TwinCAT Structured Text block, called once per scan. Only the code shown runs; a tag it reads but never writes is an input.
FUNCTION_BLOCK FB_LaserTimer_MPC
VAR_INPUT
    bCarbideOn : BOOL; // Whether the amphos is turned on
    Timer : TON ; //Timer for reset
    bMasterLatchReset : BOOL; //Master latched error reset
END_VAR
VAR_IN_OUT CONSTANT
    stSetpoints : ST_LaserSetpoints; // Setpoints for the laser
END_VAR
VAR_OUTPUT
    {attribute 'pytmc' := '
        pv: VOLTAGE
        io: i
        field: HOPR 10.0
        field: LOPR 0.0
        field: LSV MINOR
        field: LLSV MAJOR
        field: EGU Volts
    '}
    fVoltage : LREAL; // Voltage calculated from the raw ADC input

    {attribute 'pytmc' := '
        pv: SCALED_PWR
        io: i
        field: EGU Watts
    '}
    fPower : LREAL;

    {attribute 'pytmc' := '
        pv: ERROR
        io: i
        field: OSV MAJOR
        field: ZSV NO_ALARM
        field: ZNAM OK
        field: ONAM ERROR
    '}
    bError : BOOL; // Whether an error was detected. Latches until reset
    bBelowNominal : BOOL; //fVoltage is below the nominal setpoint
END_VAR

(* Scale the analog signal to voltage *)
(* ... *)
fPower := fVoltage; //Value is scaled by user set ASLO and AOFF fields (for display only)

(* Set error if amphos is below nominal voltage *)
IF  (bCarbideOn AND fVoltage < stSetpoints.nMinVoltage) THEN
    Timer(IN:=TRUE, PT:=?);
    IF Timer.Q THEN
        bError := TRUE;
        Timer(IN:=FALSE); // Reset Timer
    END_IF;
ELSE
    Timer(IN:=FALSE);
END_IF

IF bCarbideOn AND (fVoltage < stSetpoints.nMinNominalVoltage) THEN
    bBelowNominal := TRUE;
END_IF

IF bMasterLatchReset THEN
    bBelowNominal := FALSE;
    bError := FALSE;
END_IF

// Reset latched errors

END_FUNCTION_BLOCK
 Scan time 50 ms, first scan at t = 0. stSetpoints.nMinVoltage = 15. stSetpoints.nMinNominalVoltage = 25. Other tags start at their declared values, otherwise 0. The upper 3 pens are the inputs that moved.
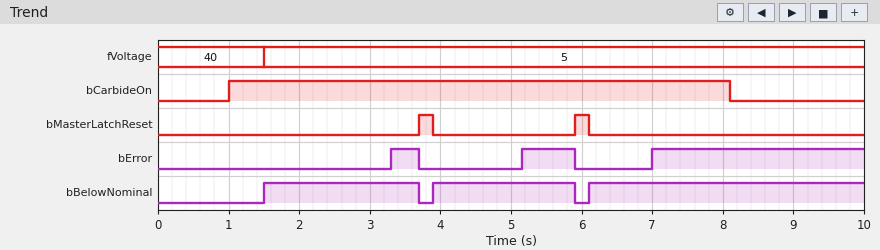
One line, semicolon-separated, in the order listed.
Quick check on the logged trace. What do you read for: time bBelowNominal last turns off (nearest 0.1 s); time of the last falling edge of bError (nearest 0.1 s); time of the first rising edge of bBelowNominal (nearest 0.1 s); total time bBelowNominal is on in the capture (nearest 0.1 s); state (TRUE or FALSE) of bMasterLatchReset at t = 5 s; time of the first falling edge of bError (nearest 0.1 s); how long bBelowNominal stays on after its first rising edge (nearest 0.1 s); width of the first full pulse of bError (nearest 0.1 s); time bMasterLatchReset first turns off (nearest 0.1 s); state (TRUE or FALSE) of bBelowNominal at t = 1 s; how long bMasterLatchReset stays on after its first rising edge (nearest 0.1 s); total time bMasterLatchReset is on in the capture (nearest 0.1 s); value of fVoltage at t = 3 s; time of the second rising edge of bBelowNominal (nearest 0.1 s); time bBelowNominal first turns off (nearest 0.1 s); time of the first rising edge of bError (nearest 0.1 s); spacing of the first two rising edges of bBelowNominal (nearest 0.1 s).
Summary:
5.9 s; 5.9 s; 1.5 s; 8.1 s; FALSE; 3.7 s; 2.2 s; 0.4 s; 3.9 s; FALSE; 0.2 s; 0.4 s; 5; 3.9 s; 3.7 s; 3.3 s; 2.4 s
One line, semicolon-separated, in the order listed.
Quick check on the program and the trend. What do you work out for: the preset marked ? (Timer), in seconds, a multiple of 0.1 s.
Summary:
1.8 s
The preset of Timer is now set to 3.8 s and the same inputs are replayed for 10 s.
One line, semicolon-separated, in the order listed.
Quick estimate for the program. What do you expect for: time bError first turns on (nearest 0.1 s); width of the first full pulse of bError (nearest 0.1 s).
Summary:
5.3 s; 0.6 s
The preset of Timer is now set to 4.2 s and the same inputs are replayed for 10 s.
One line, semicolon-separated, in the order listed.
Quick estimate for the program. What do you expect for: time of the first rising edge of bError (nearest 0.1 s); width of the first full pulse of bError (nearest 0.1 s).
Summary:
5.7 s; 0.2 s
